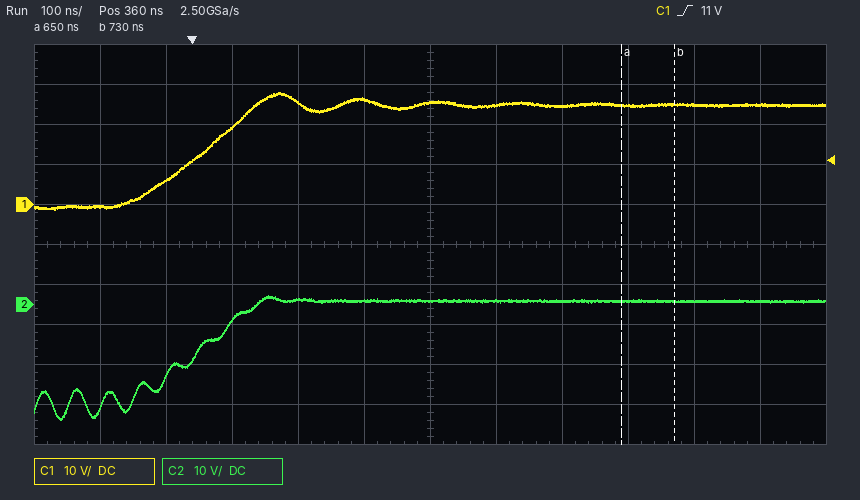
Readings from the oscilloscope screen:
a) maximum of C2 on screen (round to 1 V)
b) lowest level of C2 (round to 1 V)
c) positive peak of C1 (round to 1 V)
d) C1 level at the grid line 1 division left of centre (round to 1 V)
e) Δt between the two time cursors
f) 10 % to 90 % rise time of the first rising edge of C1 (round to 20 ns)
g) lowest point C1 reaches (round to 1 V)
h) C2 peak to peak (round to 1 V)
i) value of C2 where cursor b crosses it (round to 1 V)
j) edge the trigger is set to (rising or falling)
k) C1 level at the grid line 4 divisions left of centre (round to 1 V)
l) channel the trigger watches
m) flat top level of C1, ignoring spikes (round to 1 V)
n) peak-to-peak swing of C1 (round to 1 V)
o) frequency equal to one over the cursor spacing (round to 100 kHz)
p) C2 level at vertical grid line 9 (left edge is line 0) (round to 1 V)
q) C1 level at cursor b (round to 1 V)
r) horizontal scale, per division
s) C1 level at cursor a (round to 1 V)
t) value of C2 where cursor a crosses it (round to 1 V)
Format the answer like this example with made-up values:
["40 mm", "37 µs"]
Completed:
["2 V", "-29 V", "28 V", "26 V", "80 ns", "160 ns", "-1 V", "31 V", "1 V", "rising", "6 V", "C1", "25 V", "29 V", "12.5 MHz", "1 V", "25 V", "100 ns", "25 V", "1 V"]
